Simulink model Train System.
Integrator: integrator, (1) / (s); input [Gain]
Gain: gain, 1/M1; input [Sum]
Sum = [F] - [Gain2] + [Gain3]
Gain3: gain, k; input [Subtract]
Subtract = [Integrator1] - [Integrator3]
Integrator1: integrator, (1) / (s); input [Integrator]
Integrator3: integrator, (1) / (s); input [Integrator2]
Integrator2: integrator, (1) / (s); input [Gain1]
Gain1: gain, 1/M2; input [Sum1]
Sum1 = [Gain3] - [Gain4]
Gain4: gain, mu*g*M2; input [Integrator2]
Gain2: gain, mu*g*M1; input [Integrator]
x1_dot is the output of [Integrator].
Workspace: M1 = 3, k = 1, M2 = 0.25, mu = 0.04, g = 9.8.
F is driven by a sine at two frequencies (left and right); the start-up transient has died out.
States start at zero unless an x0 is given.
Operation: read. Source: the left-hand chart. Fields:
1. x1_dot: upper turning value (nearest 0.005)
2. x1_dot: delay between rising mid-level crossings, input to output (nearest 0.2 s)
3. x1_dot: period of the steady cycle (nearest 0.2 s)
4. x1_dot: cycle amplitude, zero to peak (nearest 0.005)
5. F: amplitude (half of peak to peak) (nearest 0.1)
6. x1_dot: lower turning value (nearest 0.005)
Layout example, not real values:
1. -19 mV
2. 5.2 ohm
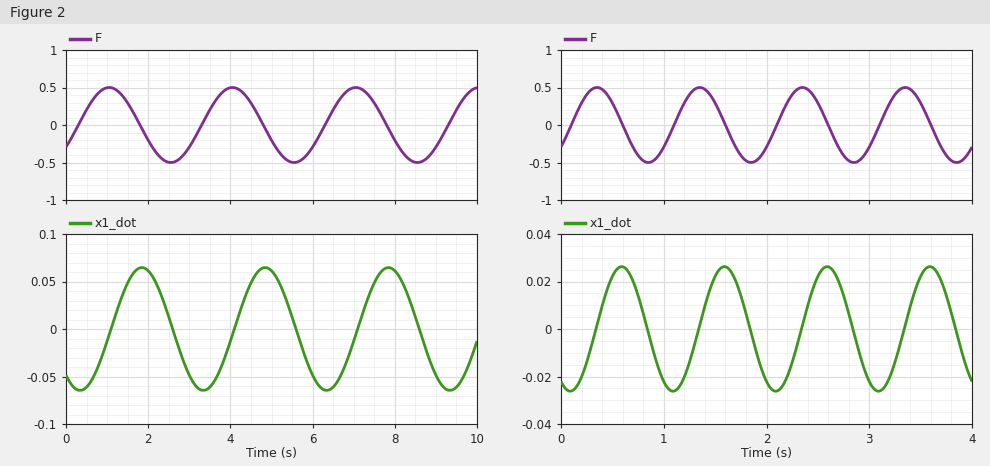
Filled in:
1. 0.065
2. 0.8 s
3. 3.0 s
4. 0.065
5. 0.5
6. -0.065
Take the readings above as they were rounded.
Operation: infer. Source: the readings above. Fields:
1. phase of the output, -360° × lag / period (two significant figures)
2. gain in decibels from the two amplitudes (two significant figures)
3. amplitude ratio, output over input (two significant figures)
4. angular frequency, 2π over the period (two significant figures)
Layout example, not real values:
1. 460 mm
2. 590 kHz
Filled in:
1. -96°
2. -18 dB
3. 0.13
4. 2.1 rad/s
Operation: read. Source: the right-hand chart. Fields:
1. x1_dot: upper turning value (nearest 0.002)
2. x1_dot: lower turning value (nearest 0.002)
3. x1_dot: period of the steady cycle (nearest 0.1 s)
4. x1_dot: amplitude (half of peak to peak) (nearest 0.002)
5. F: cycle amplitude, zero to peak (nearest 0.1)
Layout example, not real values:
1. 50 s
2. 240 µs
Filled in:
1. 0.026
2. -0.026
3. 1.0 s
4. 0.026
5. 0.5
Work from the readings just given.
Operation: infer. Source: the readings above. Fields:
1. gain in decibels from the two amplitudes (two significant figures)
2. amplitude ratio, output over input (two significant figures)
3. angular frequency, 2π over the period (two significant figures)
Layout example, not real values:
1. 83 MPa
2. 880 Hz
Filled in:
1. -26 dB
2. 0.052
3. 6.3 rad/s
